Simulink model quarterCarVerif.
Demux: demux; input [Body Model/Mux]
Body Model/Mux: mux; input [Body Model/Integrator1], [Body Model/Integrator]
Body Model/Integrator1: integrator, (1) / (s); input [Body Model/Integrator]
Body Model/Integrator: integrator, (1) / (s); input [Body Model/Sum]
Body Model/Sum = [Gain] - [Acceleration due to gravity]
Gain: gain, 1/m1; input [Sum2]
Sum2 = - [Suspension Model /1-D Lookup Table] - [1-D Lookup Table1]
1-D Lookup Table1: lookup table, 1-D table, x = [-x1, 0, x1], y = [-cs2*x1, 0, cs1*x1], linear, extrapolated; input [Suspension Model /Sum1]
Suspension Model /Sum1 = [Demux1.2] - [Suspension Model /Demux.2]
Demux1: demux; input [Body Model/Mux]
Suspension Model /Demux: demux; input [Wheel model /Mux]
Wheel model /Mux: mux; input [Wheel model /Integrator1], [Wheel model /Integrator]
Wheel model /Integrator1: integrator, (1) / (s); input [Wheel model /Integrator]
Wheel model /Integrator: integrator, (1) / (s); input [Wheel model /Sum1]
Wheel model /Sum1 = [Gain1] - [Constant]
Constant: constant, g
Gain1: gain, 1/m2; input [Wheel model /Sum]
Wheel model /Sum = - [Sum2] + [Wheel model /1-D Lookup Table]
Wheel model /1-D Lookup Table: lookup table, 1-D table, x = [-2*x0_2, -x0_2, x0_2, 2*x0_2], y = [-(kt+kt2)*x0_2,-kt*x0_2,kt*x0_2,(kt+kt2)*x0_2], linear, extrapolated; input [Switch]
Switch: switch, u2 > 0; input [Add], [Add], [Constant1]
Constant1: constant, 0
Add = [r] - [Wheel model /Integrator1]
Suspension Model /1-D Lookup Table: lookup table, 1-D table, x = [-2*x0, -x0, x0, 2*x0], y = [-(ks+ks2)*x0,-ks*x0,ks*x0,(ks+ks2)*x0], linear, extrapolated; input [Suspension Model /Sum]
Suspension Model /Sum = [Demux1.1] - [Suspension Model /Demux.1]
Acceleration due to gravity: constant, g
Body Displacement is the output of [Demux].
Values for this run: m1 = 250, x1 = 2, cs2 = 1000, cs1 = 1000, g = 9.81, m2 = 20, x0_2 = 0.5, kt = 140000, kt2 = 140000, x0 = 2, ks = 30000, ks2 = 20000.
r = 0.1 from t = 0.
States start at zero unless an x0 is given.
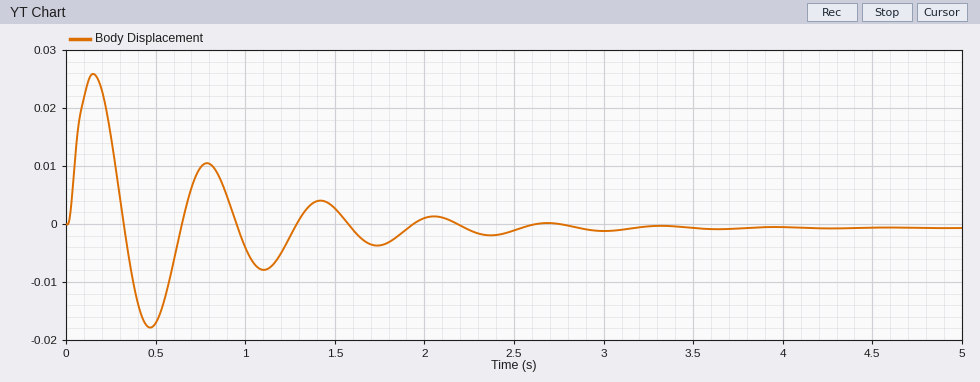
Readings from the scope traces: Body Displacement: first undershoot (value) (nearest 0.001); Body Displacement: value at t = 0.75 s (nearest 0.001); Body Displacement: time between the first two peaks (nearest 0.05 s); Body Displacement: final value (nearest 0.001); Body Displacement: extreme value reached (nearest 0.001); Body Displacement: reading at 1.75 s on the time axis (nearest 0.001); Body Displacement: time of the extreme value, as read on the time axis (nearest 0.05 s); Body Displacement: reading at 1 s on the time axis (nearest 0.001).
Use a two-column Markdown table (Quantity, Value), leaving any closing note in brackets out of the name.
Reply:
| Quantity | Value |
|---|---|
| Body Displacement: first undershoot (value) | -0.018 |
| Body Displacement: value at t = 0.75 s | 0.010 |
| Body Displacement: time between the first two peaks | 0.65 s |
| Body Displacement: final value | -0.001 |
| Body Displacement: extreme value reached | 0.026 |
| Body Displacement: reading at 1.75 s on the time axis | -0.004 |
| Body Displacement: time of the extreme value, as read on the time axis | 0.15 s |
| Body Displacement: reading at 1 s on the time axis | -0.004 |
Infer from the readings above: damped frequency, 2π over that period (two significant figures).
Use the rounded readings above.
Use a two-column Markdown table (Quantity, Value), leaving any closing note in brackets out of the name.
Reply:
| Quantity | Value |
|---|---|
| damped frequency, 2π over that period | 9.7 rad/s |
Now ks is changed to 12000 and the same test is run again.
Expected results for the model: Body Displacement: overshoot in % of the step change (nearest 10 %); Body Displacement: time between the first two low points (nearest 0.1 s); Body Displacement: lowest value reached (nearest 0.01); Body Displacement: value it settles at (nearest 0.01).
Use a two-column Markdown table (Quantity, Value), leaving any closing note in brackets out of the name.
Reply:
| Quantity | Value |
|---|---|
| Body Displacement: overshoot in % of the step change | 50 % |
| Body Displacement: time between the first two low points | 1.0 s |
| Body Displacement: lowest value reached | -0.18 |
| Body Displacement: value it settles at | -0.12 |
